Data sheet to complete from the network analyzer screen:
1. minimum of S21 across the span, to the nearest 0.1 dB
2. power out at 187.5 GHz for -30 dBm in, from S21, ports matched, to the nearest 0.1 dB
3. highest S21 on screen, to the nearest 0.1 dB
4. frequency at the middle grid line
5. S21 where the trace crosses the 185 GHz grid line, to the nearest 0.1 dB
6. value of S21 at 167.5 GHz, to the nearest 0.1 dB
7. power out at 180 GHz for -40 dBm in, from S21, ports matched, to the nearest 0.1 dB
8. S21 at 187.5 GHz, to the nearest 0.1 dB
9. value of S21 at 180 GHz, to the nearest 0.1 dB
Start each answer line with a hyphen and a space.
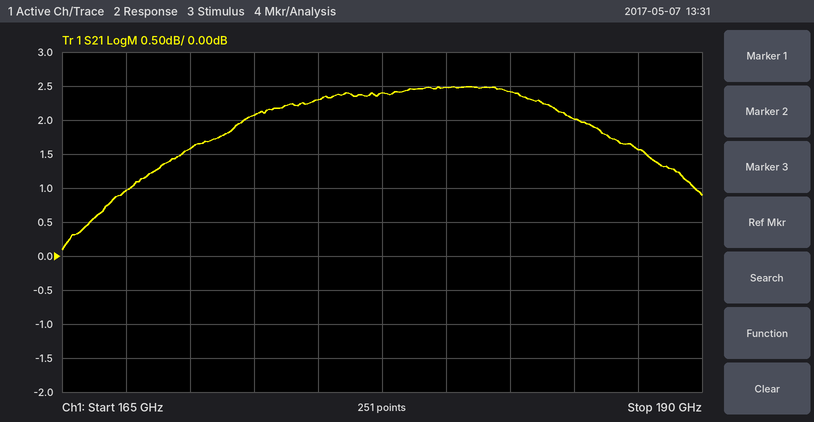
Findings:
- 0.1 dB
- -28.4 dBm
- 2.5 dB
- 177.5 GHz
- 2.0 dB
- 1.0 dB
- -37.5 dBm
- 1.6 dB
- 2.5 dB
